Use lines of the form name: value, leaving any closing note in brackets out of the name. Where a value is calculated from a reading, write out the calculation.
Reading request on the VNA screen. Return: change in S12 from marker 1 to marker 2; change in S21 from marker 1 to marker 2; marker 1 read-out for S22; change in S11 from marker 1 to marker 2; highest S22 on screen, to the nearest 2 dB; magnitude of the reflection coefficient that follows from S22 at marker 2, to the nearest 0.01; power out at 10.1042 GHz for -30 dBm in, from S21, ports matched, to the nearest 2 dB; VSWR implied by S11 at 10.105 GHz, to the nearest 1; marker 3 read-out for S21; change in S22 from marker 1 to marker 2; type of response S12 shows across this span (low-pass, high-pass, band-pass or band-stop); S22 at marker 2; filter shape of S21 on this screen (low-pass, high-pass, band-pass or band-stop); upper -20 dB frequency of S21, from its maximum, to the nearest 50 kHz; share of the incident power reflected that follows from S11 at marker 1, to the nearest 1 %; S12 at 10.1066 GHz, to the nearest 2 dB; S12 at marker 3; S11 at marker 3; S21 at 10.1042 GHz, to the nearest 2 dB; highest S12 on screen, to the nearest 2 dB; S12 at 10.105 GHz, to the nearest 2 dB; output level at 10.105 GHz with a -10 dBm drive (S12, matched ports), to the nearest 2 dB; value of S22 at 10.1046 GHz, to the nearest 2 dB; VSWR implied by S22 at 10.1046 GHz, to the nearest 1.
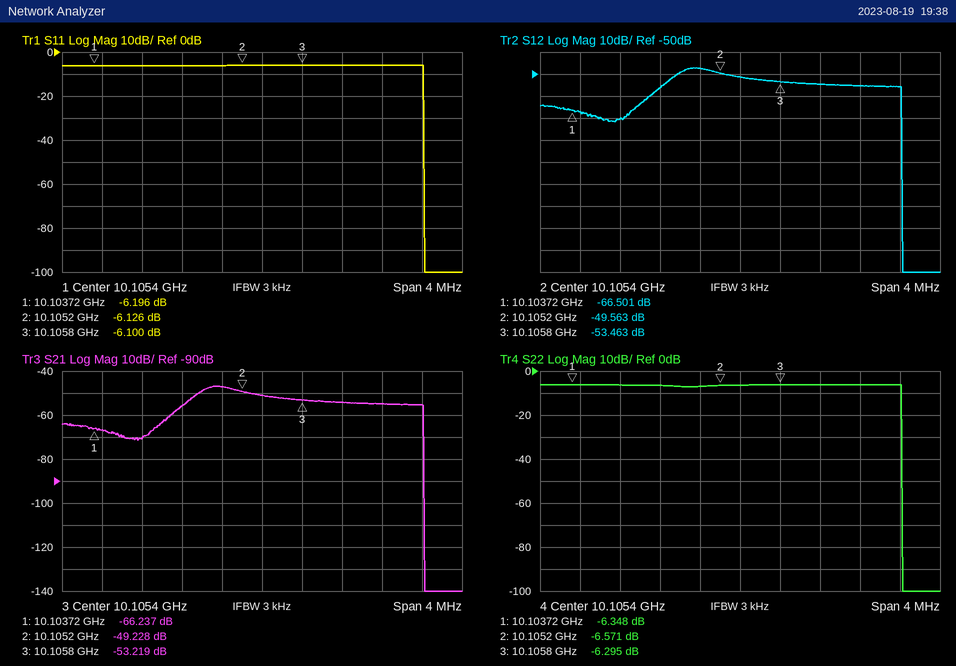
change in S12 from marker 1 to marker 2: -49.563 − (-66.501) = 16.938 dB
change in S21 from marker 1 to marker 2: -49.228 − (-66.237) = 17.009 dB
marker 1 read-out for S22: -6.348 dB
change in S11 from marker 1 to marker 2: -6.126 − (-6.196) = 0.070 dB
highest S22 on screen, to the nearest 2 dB: -6 dB
magnitude of the reflection coefficient that follows from S22 at marker 2, to the nearest 0.01: 10^(-6.571/20) ≈ 0.47
power out at 10.1042 GHz for -30 dBm in, from S21, ports matched, to the nearest 2 dB: -30 dBm + (-70 dB) = -100 dBm
VSWR implied by S11 at 10.105 GHz, to the nearest 1: |Γ| = 10^(-6/20) = 0.5012; VSWR = (1 + 0.5012)/(1 − 0.5012) ≈ 3
marker 3 read-out for S21: -53.219 dB
change in S22 from marker 1 to marker 2: -6.571 − (-6.348) = -0.223 dB
type of response S12 shows across this span: band-pass
S22 at marker 2: -6.571 dB
filter shape of S21 on this screen: band-pass
upper -20 dB frequency of S21, from its maximum, to the nearest 50 kHz: 10.10700 GHz
share of the incident power reflected that follows from S11 at marker 1, to the nearest 1 %: 10^(-6.196/10) ≈ 24 %
S12 at 10.1066 GHz, to the nearest 2 dB: -56 dB
S12 at marker 3: -53.463 dB
S11 at marker 3: -6.100 dB
S21 at 10.1042 GHz, to the nearest 2 dB: -70 dB
highest S12 on screen, to the nearest 2 dB: -48 dB
S12 at 10.105 GHz, to the nearest 2 dB: -48 dB
output level at 10.105 GHz with a -10 dBm drive (S12, matched ports), to the nearest 2 dB: -10 dBm + (-48 dB) = -58 dBm
value of S22 at 10.1046 GHz, to the nearest 2 dB: -6 dB
VSWR implied by S22 at 10.1046 GHz, to the nearest 1: |Γ| = 10^(-6/20) = 0.5012; VSWR = (1 + 0.5012)/(1 − 0.5012) ≈ 3
